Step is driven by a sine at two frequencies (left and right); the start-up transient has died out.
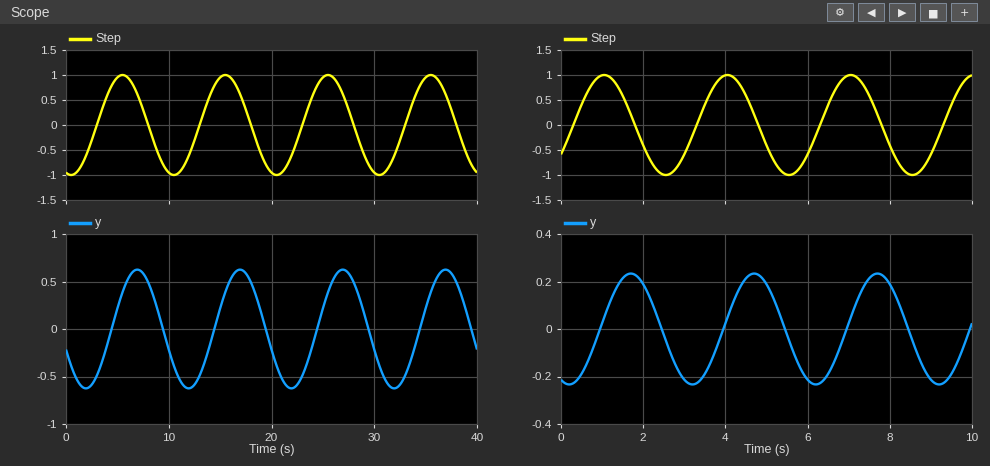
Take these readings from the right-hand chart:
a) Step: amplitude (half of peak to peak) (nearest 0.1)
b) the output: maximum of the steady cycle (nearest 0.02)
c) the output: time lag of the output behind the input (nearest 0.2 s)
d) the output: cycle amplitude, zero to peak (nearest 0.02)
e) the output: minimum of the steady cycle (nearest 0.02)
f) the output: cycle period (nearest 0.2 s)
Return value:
1.0
0.24
0.6 s
0.24
-0.24
3.0 s
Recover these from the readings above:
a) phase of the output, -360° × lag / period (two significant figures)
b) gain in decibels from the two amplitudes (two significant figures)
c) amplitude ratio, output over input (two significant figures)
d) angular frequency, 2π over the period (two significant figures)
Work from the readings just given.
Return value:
-72°
-12 dB
0.24
2.1 rad/s
